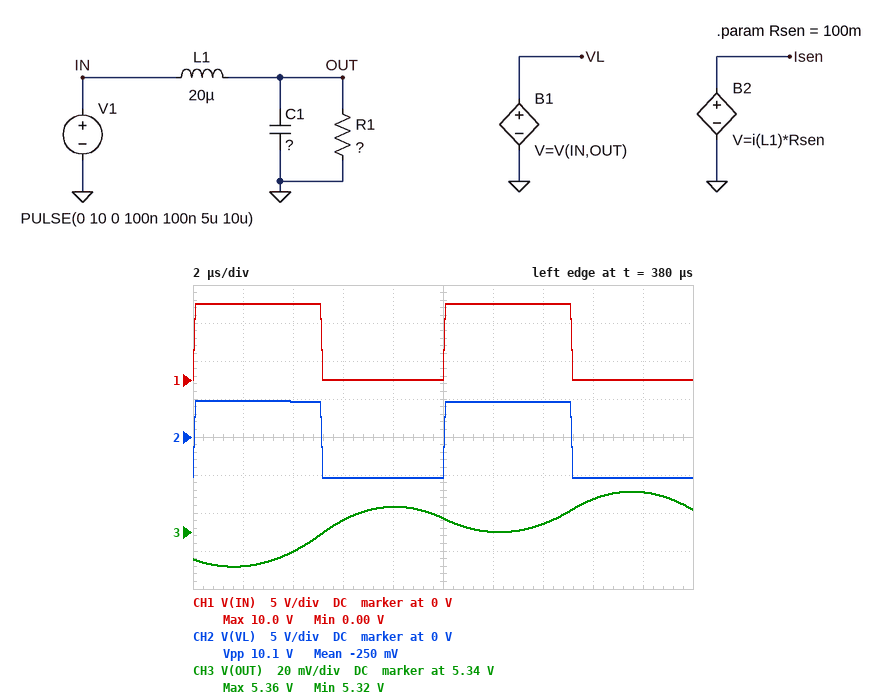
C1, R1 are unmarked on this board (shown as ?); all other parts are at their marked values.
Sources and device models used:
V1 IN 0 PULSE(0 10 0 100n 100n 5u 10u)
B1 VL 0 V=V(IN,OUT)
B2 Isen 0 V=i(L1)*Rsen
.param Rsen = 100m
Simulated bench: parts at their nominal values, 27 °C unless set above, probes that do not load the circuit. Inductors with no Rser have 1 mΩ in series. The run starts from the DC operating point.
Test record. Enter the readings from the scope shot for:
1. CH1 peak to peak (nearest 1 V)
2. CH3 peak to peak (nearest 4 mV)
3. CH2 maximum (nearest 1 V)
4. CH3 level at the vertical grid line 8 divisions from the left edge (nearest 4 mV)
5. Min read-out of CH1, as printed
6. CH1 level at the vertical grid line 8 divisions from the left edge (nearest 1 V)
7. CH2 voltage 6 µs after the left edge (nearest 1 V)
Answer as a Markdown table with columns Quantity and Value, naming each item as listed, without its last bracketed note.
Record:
| Quantity | Value |
|---|---|
| CH1 peak to peak | 10 V |
| CH3 peak to peak | 40 mV |
| CH2 maximum | 5 V |
| CH3 level at the vertical grid line 8 divisions from the left edge | 5.356 V |
| Min read-out of CH1, as printed | 0.00 V |
| CH1 level at the vertical grid line 8 divisions from the left edge | 0 V |
| CH2 voltage 6 µs after the left edge | -5 V |
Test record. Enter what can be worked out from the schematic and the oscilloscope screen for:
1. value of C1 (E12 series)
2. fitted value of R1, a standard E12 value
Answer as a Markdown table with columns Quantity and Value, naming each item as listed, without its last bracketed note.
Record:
| Quantity | Value |
|---|---|
| value of C1 | 82 µF |
| fitted value of R1, a standard E12 value | 0.82 Ω |
